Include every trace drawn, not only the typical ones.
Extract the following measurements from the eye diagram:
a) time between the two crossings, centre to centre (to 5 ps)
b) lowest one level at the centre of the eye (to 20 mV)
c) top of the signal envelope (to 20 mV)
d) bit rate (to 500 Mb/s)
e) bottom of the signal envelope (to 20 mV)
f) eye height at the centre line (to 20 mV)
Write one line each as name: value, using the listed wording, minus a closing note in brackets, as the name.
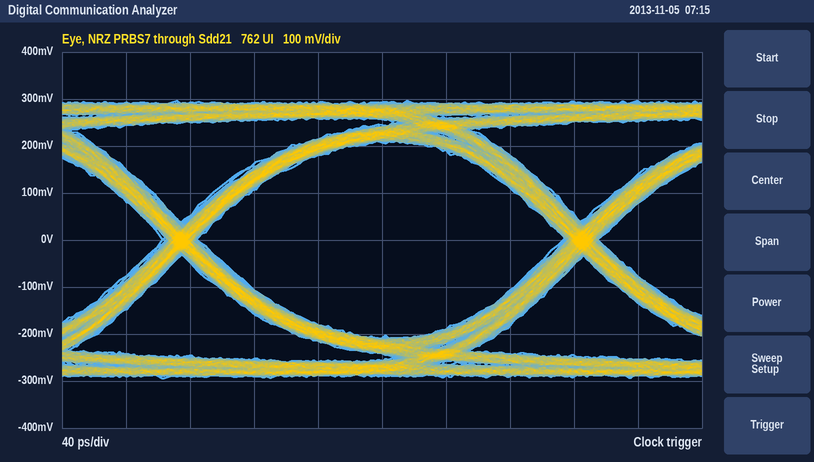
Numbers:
time between the two crossings, centre to centre: 250 ps
lowest one level at the centre of the eye: 200 mV
top of the signal envelope: 300 mV
bit rate: 4.0 Gb/s
bottom of the signal envelope: -300 mV
eye height at the centre line: 420 mV
